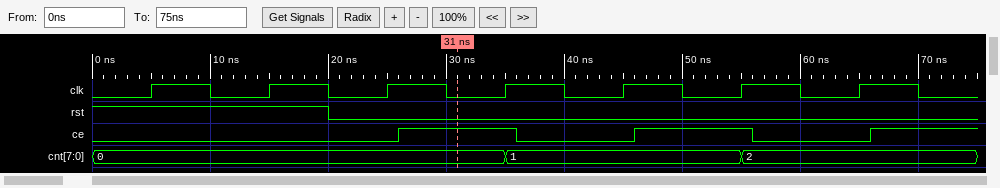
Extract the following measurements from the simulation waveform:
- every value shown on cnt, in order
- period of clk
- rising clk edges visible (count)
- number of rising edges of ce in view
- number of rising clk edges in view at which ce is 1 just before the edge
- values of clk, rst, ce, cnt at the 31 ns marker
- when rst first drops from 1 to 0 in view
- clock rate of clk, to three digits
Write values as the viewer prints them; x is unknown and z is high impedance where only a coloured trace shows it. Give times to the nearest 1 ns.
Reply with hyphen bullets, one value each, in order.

- 0, 1, 2
- 10 ns
- 7
- 3
- 2
- clk=0, rst=0, ce=1, cnt=0
- 20 ns
- 100 MHz
